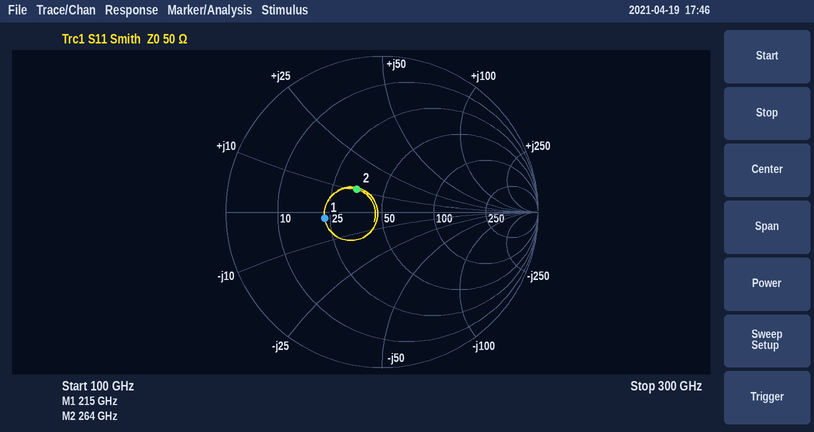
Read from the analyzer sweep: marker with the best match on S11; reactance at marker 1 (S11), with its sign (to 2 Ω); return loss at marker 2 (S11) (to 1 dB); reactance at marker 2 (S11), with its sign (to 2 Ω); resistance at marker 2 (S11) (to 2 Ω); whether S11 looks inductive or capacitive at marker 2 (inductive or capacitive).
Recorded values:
marker 2
-2 Ω
13 dB
+10 Ω
34 Ω
inductive
